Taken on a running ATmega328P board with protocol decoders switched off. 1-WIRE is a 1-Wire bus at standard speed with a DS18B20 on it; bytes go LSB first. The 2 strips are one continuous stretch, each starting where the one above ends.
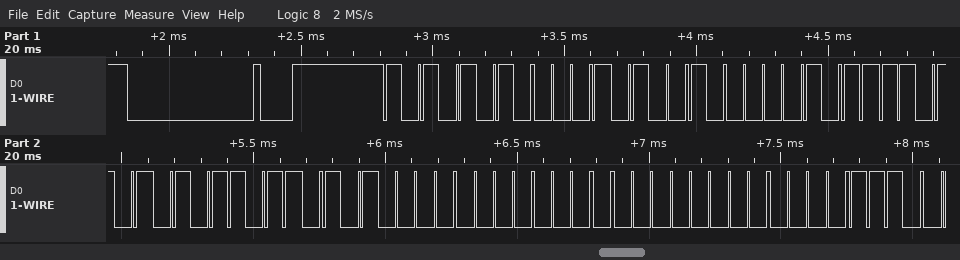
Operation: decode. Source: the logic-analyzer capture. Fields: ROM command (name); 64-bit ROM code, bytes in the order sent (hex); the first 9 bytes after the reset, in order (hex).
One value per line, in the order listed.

Match ROM
28 41 AF DA 0A 00 00 70
55 28 41 AF DA 0A 00 00 70
